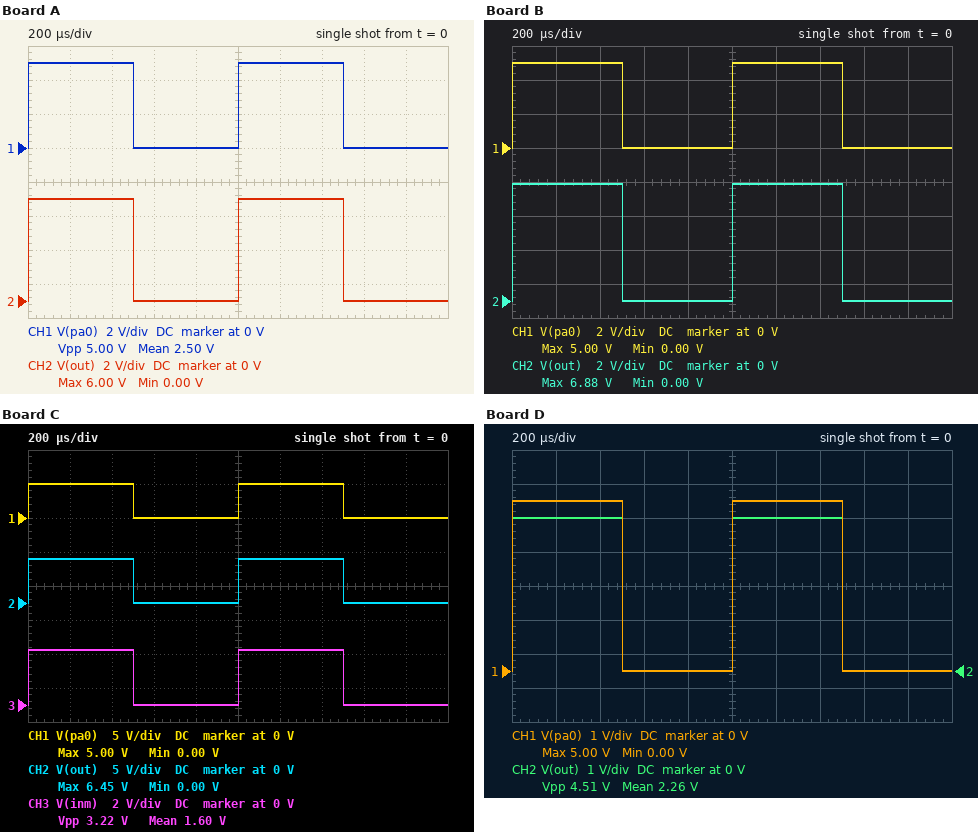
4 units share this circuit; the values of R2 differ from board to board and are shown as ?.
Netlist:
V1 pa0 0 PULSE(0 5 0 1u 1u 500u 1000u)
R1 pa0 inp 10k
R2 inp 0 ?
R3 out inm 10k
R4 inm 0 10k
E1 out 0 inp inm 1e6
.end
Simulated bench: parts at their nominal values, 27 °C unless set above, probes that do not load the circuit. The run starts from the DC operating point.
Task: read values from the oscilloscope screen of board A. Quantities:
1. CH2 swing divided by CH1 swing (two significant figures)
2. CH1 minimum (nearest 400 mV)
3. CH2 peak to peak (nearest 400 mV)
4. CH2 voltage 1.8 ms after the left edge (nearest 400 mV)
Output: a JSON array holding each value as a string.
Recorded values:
["1.2", "0 V", "6.0 V", "0 V"]
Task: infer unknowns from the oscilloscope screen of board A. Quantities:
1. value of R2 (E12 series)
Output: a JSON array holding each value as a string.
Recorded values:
["15 kΩ"]
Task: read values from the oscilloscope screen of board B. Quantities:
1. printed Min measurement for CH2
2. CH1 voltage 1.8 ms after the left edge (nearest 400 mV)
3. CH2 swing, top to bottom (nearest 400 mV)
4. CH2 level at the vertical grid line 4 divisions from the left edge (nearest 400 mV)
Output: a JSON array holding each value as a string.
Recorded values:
["0.00 V", "0 V", "6.8 V", "0 V"]
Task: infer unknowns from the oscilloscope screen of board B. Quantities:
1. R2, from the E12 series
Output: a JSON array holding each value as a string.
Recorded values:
["22 kΩ"]
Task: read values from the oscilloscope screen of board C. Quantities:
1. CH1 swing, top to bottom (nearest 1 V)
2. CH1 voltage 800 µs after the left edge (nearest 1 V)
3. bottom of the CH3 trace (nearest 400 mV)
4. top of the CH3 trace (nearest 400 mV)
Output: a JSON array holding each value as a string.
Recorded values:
["5 V", "0 V", "0 V", "3.2 V"]
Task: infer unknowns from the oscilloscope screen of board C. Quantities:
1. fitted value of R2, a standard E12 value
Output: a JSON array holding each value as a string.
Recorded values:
["18 kΩ"]
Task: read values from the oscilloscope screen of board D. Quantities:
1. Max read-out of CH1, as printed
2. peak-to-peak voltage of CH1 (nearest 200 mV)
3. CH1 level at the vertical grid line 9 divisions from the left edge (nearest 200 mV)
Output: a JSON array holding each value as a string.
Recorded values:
["5.00 V", "5.0 V", "0 V"]
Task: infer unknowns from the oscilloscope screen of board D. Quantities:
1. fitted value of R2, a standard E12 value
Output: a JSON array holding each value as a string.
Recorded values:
["8.2 kΩ"]
